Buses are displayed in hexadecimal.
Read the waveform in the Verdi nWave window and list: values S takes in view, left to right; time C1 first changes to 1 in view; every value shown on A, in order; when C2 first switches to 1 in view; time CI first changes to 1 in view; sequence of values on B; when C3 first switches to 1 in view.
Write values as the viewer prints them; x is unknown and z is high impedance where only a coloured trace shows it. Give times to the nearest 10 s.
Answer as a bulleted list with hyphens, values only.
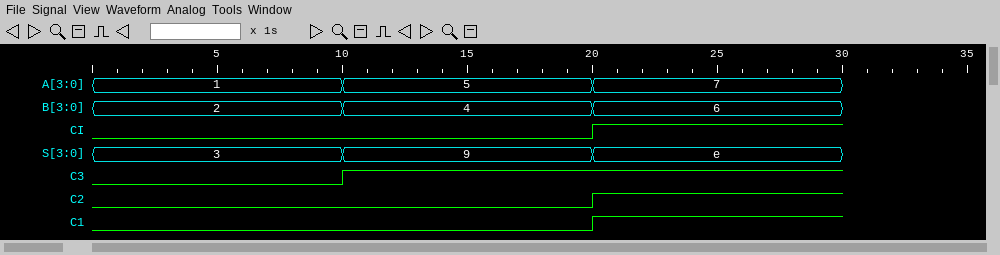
- 3, 9, e
- 20 s
- 1, 5, 7
- 20 s
- 20 s
- 2, 4, 6
- 10 s
